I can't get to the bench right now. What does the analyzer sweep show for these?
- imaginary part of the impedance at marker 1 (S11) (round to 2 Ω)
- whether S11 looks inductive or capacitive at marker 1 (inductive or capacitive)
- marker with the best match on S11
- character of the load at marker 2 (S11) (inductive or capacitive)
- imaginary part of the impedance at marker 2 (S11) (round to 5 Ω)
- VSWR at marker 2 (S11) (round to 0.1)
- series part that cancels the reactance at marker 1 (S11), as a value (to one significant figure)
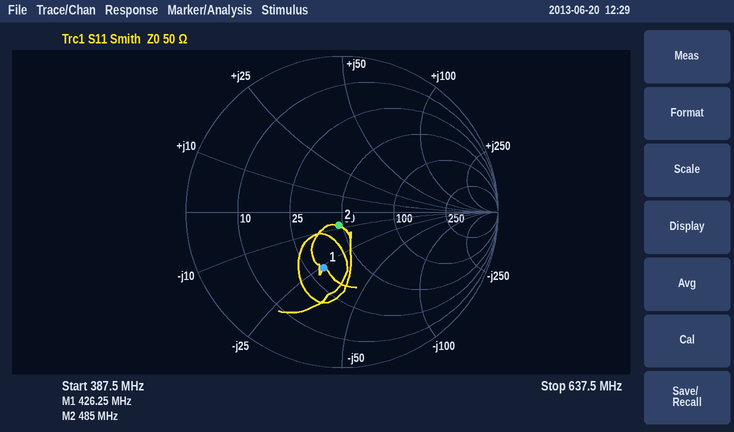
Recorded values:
-26 Ω
capacitive
marker 2
capacitive
-10 Ω
1.2
10 nH
